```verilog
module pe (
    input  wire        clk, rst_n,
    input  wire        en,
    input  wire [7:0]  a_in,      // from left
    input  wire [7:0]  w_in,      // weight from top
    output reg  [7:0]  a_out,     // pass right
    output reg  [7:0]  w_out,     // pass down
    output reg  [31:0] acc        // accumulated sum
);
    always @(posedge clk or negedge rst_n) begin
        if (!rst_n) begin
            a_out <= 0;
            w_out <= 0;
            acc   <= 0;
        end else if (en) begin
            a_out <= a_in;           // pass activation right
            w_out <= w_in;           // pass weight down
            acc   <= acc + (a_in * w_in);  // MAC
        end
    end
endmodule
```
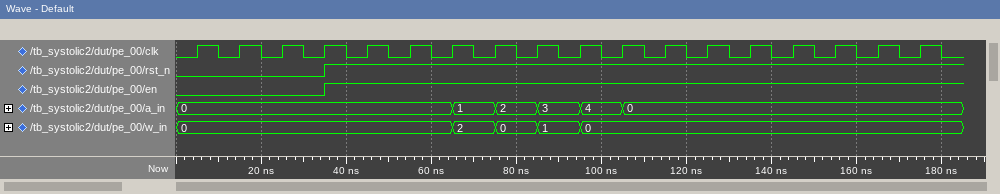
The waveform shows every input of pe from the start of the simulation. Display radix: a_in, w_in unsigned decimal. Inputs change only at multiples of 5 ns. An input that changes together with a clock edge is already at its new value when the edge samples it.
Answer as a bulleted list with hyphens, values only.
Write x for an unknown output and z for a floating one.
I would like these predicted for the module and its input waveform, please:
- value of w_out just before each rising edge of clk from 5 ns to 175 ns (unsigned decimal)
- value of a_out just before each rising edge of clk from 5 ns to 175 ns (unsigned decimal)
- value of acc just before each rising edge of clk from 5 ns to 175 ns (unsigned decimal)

- 0, 0, 0, 0, 0, 0, 0, 2, 0, 1, 0, 0, 0, 0, 0, 0, 0, 0
- 0, 0, 0, 0, 0, 0, 0, 1, 2, 3, 4, 0, 0, 0, 0, 0, 0, 0
- 0, 0, 0, 0, 0, 0, 0, 2, 2, 5, 5, 5, 5, 5, 5, 5, 5, 5
